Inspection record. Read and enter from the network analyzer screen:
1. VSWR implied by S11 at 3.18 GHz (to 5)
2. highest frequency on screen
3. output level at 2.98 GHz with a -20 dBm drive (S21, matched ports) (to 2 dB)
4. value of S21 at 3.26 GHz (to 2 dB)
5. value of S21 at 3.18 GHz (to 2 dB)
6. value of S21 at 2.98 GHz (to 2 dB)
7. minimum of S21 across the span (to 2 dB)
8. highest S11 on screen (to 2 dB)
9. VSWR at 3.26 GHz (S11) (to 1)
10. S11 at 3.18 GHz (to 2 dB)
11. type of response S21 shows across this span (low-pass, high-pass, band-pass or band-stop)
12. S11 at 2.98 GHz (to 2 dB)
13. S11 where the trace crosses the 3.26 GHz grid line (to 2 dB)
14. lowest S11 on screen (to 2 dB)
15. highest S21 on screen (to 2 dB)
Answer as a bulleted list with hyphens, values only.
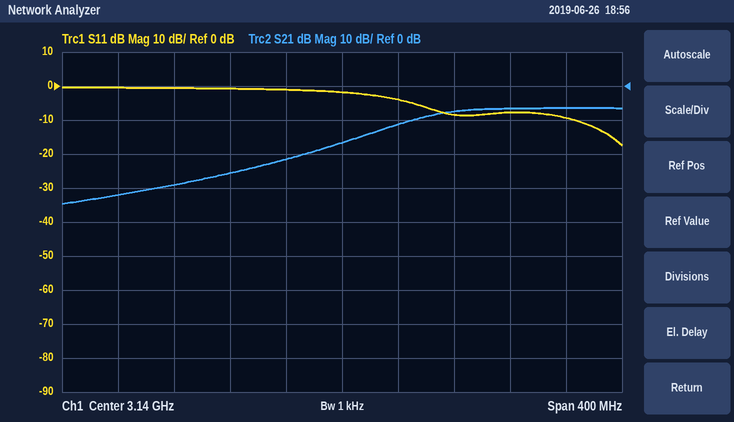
- 5
- 3.34 GHz
- -52 dBm
- -6 dB
- -12 dB
- -32 dB
- -34 dB
- 0 dB
- 2
- -4 dB
- high-pass
- 0 dB
- -8 dB
- -18 dB
- -6 dB
